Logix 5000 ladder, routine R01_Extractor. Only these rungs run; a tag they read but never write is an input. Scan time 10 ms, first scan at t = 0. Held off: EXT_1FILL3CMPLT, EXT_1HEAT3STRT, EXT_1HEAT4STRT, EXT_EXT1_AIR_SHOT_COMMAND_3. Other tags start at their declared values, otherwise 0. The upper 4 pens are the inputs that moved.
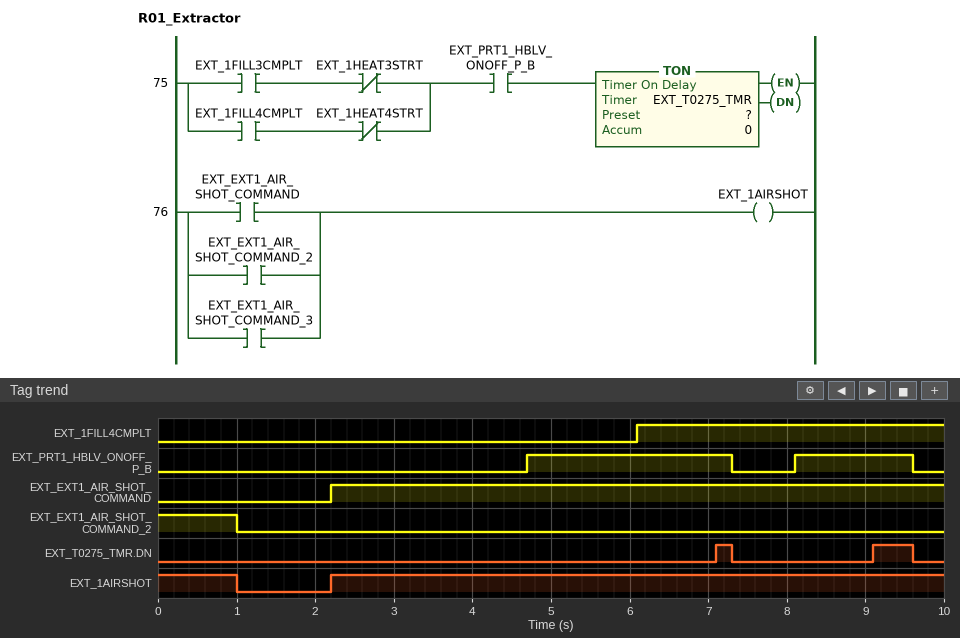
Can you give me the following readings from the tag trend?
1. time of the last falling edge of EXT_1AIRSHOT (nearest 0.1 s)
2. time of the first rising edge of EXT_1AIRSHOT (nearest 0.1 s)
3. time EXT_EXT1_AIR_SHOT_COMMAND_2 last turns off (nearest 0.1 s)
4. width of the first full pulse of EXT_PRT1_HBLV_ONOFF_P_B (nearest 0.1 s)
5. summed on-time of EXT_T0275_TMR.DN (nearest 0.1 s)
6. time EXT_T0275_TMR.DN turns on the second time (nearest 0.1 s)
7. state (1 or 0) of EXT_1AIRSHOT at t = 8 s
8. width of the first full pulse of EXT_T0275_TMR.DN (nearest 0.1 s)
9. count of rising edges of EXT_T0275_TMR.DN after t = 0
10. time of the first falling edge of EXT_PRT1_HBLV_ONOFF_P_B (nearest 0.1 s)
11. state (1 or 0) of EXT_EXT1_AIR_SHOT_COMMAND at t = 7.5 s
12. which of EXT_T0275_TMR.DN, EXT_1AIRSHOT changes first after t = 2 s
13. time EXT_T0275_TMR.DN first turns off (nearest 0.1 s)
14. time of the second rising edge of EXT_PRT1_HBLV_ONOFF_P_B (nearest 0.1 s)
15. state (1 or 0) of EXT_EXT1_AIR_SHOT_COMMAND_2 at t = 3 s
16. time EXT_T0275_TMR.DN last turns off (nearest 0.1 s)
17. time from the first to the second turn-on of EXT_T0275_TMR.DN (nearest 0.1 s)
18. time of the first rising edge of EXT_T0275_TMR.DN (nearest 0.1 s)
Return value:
1.0 s
2.2 s
1.0 s
2.6 s
0.7 s
9.1 s
1
0.2 s
2
7.3 s
1
EXT_1AIRSHOT
7.3 s
8.1 s
0
9.6 s
2.0 s
7.1 s
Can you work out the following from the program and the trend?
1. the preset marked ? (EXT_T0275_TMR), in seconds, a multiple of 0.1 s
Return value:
1.0 s
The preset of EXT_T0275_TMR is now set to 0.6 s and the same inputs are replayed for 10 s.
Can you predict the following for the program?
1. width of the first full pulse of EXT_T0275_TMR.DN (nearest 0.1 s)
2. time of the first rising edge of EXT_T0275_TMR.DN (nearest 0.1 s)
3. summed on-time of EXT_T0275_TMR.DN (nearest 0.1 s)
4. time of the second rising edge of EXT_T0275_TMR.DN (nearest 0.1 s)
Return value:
0.6 s
6.7 s
1.5 s
8.7 s
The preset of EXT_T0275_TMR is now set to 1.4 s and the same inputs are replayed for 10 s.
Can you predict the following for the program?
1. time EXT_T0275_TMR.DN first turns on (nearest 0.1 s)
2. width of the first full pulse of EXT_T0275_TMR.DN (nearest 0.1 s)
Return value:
9.5 s
0.1 s
